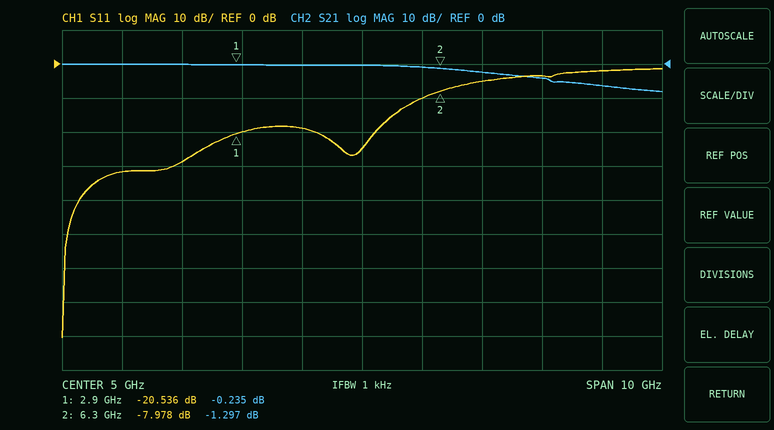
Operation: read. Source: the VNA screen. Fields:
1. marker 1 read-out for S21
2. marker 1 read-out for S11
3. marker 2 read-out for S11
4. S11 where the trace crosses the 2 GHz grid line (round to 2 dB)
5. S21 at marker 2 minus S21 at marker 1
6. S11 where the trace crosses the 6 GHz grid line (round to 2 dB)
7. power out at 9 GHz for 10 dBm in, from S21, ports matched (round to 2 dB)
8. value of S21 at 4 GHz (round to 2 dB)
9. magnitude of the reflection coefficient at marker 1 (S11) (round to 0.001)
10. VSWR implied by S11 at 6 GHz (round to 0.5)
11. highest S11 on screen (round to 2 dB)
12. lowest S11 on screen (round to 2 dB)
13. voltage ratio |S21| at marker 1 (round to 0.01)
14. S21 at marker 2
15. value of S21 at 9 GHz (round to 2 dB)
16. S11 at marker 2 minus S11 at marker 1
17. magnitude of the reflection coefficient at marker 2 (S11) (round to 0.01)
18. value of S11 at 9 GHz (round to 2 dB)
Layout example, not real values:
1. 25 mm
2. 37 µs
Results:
1. -0.235 dB
2. -20.536 dB
3. -7.978 dB
4. -28 dB
5. -1.062 dB
6. -10 dB
7. 4 dBm
8. 0 dB
9. 0.094
10. 2.0
11. -2 dB
12. -80 dB
13. 0.97
14. -1.297 dB
15. -6 dB
16. 12.558 dB
17. 0.40
18. -2 dB
